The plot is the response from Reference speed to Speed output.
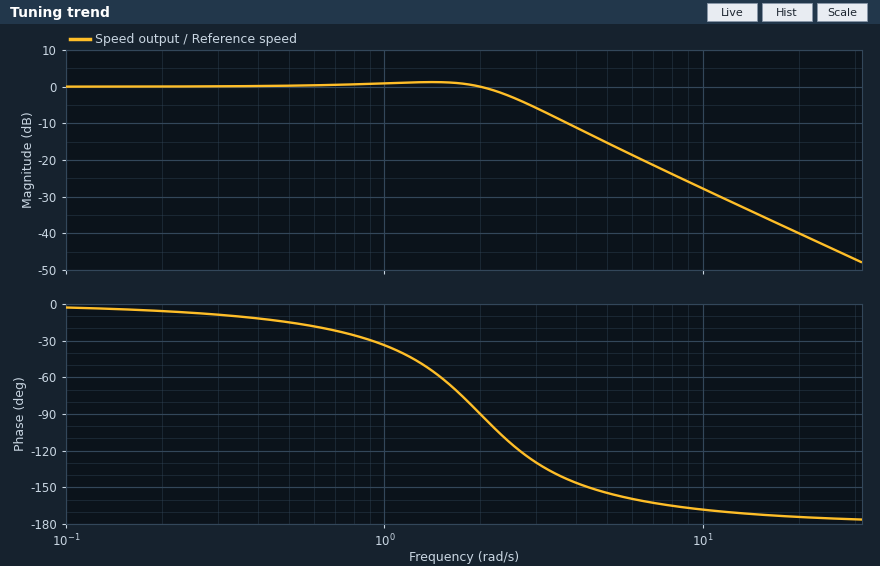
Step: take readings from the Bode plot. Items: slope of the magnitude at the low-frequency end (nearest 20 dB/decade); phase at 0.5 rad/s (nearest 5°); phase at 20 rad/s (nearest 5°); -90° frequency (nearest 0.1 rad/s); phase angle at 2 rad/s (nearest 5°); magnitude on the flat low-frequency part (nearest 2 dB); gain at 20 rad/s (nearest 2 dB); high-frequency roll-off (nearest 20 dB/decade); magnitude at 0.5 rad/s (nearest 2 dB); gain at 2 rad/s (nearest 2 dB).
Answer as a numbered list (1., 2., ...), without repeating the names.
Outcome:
1. 0 dB/decade
2. -15°
3. -175°
4. 2.0 rad/s
5. -90°
6. 0 dB
7. -40 dB
8. -40 dB/decade
9. 0 dB
10. 0 dB
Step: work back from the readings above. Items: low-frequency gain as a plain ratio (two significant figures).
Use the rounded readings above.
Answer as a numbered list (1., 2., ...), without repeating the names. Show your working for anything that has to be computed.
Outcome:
1. 10^(0 / 20) = 1.0
